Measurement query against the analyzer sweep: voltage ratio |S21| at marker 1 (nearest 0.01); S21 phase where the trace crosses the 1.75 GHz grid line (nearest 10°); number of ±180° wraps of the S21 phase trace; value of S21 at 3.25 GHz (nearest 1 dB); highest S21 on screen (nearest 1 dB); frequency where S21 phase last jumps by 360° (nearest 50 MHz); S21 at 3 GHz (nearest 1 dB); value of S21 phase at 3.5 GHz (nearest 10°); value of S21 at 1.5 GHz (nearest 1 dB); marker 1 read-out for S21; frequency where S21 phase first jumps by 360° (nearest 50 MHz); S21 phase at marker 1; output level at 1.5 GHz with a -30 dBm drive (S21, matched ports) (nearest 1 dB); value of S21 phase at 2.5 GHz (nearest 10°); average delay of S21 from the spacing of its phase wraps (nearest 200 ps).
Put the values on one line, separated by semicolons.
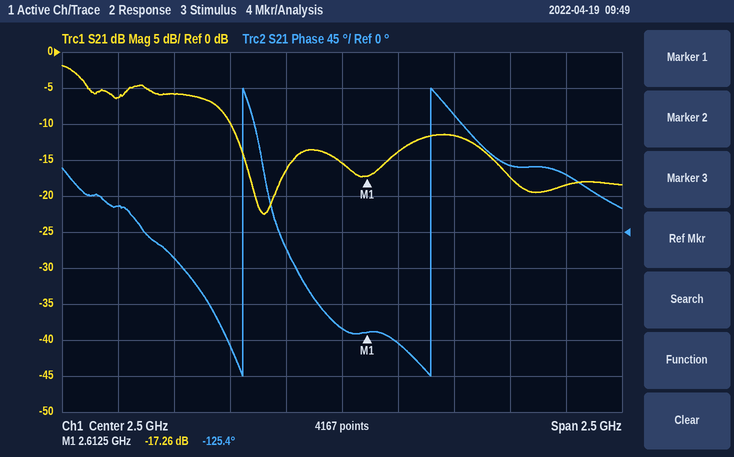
0.14; -30°; 2; -17 dB; -2 dB; 2.90 GHz; -12 dB; 70°; -6 dB; -17.26 dB; 2.05 GHz; -125.4°; -36 dBm; -120°; 1.2 ns
